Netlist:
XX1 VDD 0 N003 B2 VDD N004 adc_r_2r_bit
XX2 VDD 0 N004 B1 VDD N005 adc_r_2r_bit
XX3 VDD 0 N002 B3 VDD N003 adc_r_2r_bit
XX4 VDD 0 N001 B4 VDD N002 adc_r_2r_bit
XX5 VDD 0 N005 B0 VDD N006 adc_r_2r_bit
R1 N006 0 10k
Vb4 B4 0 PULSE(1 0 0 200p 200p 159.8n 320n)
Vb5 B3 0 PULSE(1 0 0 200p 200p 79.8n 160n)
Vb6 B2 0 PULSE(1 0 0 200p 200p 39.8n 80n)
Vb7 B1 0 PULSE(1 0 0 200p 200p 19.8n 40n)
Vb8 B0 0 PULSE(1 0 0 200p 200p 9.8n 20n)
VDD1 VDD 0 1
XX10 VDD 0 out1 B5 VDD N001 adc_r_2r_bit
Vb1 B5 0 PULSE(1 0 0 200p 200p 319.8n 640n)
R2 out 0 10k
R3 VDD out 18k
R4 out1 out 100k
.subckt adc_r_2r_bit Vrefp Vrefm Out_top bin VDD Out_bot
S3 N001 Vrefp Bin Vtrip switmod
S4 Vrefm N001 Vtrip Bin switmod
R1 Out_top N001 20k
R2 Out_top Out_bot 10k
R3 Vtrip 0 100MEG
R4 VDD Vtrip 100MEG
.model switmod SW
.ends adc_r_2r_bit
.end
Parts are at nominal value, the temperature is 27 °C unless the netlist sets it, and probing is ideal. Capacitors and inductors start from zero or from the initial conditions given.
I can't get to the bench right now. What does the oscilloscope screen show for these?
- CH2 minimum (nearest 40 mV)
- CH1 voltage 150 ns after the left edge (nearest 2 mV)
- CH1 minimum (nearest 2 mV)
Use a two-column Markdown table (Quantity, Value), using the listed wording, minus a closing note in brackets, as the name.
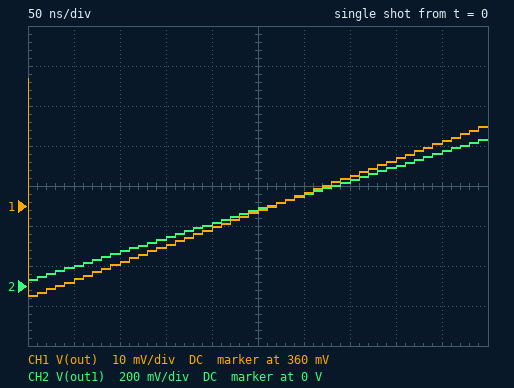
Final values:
| Quantity | Value |
|---|---|
| CH2 minimum | 40 mV |
| CH1 voltage 150 ns after the left edge | 350 mV |
| CH1 minimum | 338 mV |
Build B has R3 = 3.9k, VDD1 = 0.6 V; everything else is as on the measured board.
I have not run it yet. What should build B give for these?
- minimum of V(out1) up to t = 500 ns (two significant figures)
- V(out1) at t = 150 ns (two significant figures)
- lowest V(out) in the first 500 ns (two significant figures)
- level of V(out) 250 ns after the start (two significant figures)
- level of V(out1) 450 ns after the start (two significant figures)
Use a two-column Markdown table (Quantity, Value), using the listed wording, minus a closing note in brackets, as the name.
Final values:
| Quantity | Value |
|---|---|
| minimum of V(out1) up to t = 500 ns | 38 mV |
| V(out1) at t = 150 ns | 160 mV |
| lowest V(out) in the first 500 ns | 420 mV |
| level of V(out) 250 ns after the start | 430 mV |
| level of V(out1) 450 ns after the start | 410 mV |
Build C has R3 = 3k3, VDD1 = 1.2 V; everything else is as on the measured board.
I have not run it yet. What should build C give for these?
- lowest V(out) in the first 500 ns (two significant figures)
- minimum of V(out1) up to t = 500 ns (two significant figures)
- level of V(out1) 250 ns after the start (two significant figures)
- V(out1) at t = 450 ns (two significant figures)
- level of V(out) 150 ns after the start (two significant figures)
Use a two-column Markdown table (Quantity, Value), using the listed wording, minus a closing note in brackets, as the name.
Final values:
| Quantity | Value |
|---|---|
| lowest V(out) in the first 500 ns | 880 mV |
| minimum of V(out1) up to t = 500 ns | 80 mV |
| level of V(out1) 250 ns after the start | 490 mV |
| V(out1) at t = 450 ns | 830 mV |
| level of V(out) 150 ns after the start | 890 mV |
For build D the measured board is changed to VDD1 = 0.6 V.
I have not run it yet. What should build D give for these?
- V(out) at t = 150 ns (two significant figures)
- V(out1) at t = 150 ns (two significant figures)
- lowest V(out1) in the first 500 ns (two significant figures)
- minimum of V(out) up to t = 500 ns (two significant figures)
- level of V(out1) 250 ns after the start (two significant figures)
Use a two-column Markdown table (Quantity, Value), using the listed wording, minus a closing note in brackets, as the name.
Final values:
| Quantity | Value |
|---|---|
| V(out) at t = 150 ns | 210 mV |
| V(out1) at t = 150 ns | 140 mV |
| lowest V(out1) in the first 500 ns | 18 mV |
| minimum of V(out) up to t = 500 ns | 200 mV |
| level of V(out1) 250 ns after the start | 220 mV |
